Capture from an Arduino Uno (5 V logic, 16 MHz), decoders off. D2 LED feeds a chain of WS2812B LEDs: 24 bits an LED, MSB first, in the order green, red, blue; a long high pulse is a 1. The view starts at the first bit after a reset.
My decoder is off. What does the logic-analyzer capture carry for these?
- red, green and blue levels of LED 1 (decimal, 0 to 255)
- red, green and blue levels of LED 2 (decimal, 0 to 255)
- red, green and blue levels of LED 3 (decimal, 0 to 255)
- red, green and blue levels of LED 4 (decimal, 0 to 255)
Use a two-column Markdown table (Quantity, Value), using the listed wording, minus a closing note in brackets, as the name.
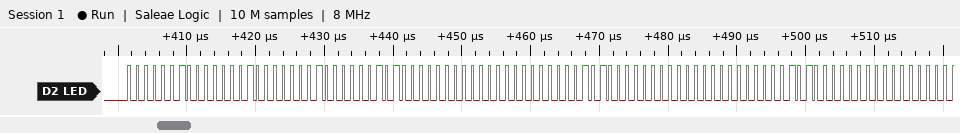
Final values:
| Quantity | Value |
|---|---|
| red, green and blue levels of LED 1 | 2, 2, 2 |
| red, green and blue levels of LED 2 | 0, 5, 0 |
| red, green and blue levels of LED 3 | 0, 5, 0 |
| red, green and blue levels of LED 4 | 0, 5, 0 |
